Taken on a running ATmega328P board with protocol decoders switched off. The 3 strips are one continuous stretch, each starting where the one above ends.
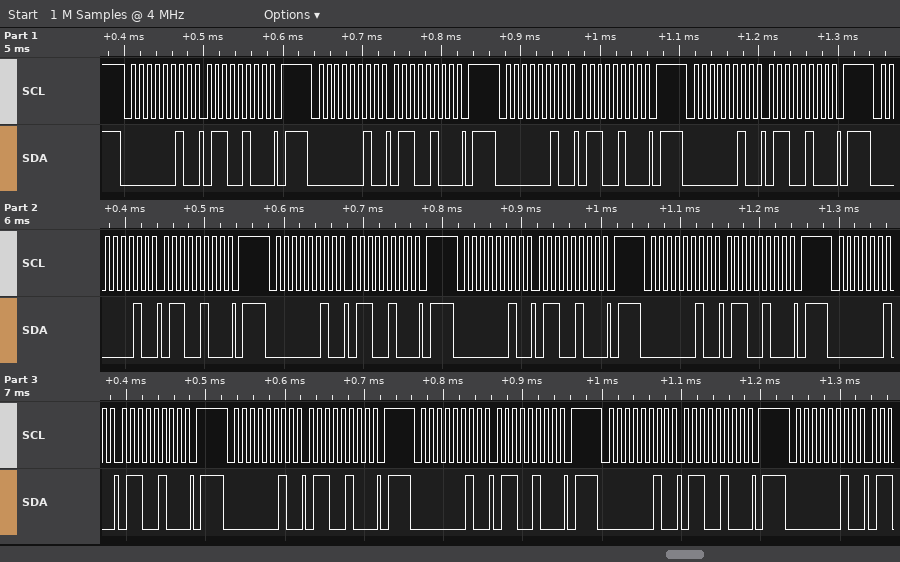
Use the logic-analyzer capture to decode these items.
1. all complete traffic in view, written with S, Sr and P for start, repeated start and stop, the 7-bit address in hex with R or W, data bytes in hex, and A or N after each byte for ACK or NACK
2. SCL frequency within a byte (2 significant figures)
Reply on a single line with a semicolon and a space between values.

S 01W A 64 A P S 01W A 64 A P S 01W A 64 A P S 01W A 64 A P S 01W A 64 A P S 01W A 64 A P S 01W A 64 A P S 01W A 64 A P S 01W A 64 A P S 01W A 64 A P S 01W A 64 A P S 01W A 64 A P S 01W A; 100 kHz
